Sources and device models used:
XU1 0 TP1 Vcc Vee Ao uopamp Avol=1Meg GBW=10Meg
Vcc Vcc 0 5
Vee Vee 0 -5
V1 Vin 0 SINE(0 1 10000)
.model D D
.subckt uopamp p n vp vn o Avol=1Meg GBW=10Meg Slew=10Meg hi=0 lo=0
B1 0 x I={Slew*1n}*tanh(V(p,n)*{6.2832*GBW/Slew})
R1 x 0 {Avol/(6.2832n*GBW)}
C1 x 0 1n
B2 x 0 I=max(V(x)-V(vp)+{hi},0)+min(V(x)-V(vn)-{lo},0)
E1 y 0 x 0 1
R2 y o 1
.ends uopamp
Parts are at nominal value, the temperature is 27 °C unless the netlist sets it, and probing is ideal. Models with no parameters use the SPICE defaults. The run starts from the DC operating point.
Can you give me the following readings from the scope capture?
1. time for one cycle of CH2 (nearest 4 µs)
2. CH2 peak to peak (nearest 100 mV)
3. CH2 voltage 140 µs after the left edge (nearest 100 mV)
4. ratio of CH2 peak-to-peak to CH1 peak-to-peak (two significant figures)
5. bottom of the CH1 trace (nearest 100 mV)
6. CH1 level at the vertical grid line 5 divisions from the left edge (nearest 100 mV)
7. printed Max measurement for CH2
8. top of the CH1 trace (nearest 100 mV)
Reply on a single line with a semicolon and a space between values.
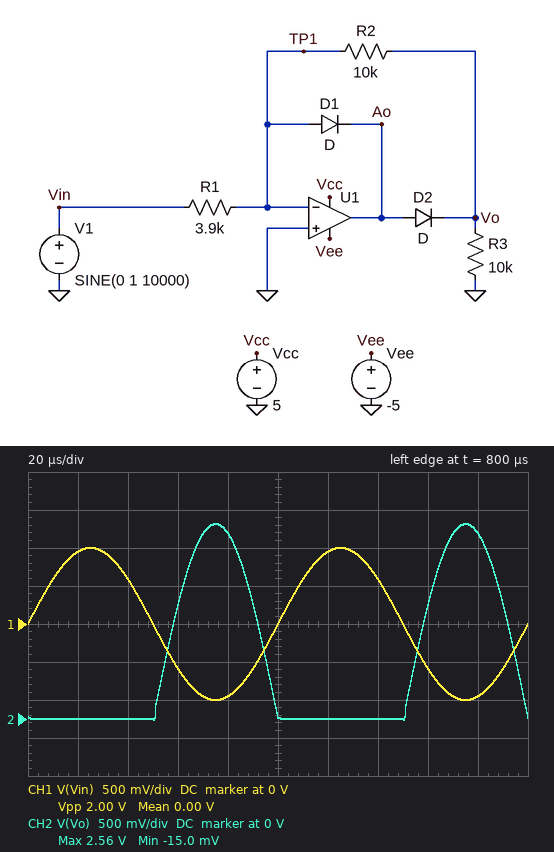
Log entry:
100 µs; 2.6 V; 0 V; 1.3; -1.0 V; 0 V; 2.56 V; 1.0 V
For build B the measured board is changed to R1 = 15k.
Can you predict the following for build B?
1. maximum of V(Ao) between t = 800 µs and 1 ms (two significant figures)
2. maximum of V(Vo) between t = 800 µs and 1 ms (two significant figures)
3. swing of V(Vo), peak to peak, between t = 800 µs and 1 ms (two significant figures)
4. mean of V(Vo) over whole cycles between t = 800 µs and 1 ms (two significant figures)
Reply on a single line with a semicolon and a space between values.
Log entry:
1.3 V; 670 mV; 680 mV; 210 mV
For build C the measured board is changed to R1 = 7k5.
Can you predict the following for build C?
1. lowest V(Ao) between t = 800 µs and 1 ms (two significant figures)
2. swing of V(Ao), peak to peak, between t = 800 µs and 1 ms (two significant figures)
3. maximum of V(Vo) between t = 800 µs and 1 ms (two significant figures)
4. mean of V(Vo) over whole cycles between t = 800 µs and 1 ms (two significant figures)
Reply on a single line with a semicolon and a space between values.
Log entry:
-600 mV; 2.6 V; 1.3 V; 420 mV
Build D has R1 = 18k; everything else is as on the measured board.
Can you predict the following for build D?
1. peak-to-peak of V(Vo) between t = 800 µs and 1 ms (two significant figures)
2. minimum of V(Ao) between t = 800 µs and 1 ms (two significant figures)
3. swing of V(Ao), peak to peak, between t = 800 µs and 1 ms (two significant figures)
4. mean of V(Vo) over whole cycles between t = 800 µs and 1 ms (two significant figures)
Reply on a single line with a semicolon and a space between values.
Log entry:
570 mV; -580 mV; 1.7 V; 180 mV
